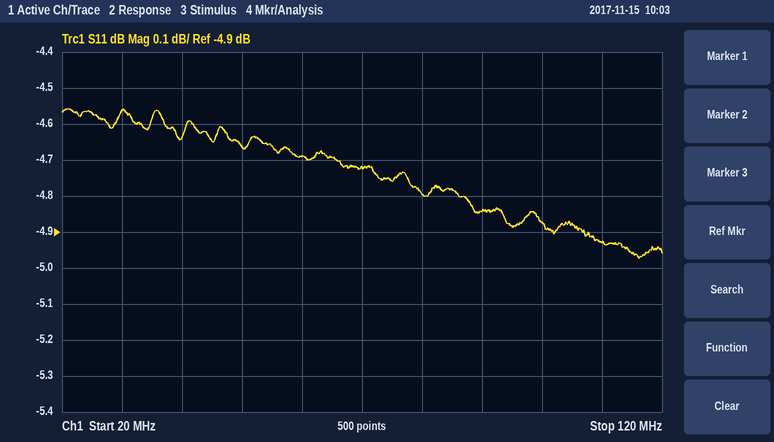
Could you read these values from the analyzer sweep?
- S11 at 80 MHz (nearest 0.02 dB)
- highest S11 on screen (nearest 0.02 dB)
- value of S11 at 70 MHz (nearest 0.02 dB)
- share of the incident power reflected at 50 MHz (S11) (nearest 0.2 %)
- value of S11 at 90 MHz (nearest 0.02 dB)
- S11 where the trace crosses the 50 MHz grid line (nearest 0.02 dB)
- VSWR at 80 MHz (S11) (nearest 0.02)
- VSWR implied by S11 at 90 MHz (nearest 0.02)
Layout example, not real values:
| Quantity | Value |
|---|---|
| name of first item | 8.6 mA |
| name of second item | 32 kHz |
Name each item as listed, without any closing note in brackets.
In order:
| Quantity | Value |
|---|---|
| S11 at 80 MHz | -4.80 dB |
| highest S11 on screen | -4.56 dB |
| value of S11 at 70 MHz | -4.72 dB |
| share of the incident power reflected at 50 MHz (S11) | 34.2 % |
| value of S11 at 90 MHz | -4.84 dB |
| S11 where the trace crosses the 50 MHz grid line | -4.66 dB |
| VSWR at 80 MHz (S11) | 3.72 |
| VSWR implied by S11 at 90 MHz | 3.68 |
